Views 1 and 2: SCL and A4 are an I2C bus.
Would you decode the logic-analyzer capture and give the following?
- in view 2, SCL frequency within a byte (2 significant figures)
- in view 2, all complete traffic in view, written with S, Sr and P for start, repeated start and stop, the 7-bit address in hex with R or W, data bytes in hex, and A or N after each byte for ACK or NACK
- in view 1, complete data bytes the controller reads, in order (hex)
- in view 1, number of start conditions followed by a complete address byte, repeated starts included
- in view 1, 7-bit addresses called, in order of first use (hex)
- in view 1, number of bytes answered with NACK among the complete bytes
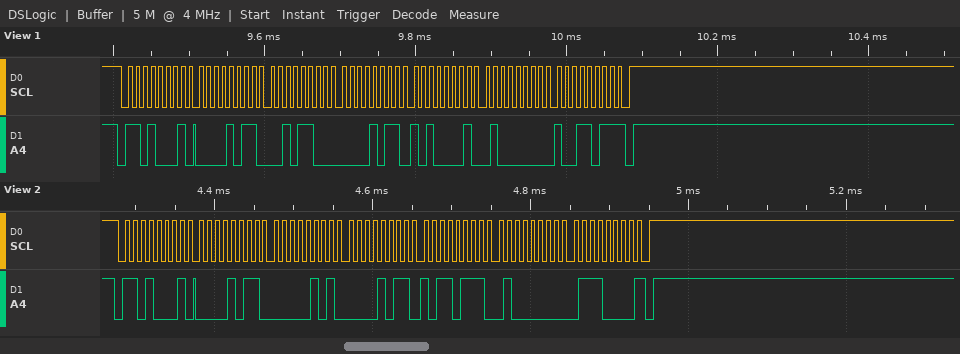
100 kHz
S 68R A 0B A 05 A 0B A B7 A 40 A 70 N P
0B 2C 0B A1 40 9B
1
0x68
1
